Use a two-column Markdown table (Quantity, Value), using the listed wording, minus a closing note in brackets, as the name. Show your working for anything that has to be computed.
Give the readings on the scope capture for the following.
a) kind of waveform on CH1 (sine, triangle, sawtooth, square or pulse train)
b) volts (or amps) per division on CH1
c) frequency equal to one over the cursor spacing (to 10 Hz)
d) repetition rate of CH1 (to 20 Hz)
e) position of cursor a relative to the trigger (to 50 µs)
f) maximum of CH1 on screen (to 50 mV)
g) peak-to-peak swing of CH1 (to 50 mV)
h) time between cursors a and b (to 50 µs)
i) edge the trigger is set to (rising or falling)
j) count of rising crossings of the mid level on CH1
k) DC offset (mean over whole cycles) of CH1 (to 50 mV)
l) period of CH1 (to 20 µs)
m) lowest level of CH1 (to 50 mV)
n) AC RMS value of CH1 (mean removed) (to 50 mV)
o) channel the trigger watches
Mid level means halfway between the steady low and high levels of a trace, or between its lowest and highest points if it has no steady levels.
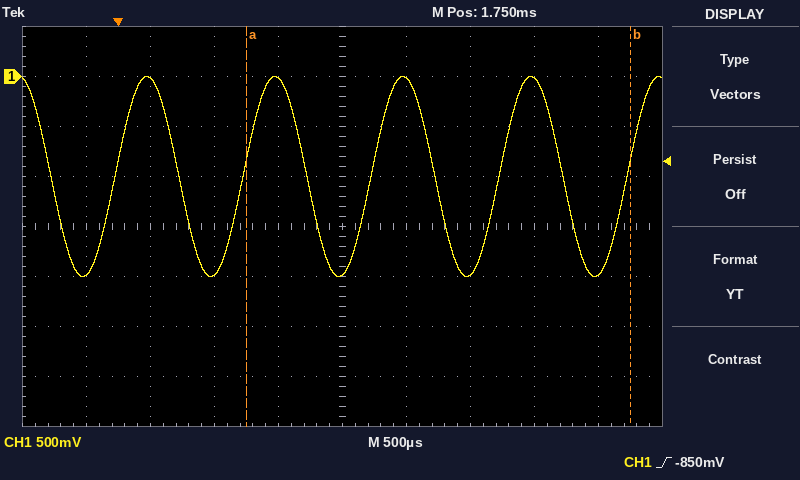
| Quantity | Value |
|---|---|
| kind of waveform on CH1 | sine |
| volts (or amps) per division on CH1 | 500 mV |
| frequency equal to one over the cursor spacing | 1 / 3.00 ms ≈ 330 Hz |
| repetition rate of CH1 | 1 / 1.00 ms ≈ 1.00 kHz |
| position of cursor a relative to the trigger | +1.00 ms |
| maximum of CH1 on screen | 0 mV |
| peak-to-peak swing of CH1 | 0 mV − (-2.00 V) = 2.00 V |
| time between cursors a and b | 3.00 ms |
| edge the trigger is set to | rising |
| count of rising crossings of the mid level on CH1 | 5 |
| DC offset (mean over whole cycles) of CH1 | (0 mV + (-2.00 V)) / 2 ≈ -1.00 V |
| period of CH1 | 1.00 ms |
| lowest level of CH1 | -2.00 V |
| AC RMS value of CH1 (mean removed) | 2.00 V / (2√2) ≈ 707 mV, so 700 mV to the nearest 50 mV |
| channel the trigger watches | CH1 |
